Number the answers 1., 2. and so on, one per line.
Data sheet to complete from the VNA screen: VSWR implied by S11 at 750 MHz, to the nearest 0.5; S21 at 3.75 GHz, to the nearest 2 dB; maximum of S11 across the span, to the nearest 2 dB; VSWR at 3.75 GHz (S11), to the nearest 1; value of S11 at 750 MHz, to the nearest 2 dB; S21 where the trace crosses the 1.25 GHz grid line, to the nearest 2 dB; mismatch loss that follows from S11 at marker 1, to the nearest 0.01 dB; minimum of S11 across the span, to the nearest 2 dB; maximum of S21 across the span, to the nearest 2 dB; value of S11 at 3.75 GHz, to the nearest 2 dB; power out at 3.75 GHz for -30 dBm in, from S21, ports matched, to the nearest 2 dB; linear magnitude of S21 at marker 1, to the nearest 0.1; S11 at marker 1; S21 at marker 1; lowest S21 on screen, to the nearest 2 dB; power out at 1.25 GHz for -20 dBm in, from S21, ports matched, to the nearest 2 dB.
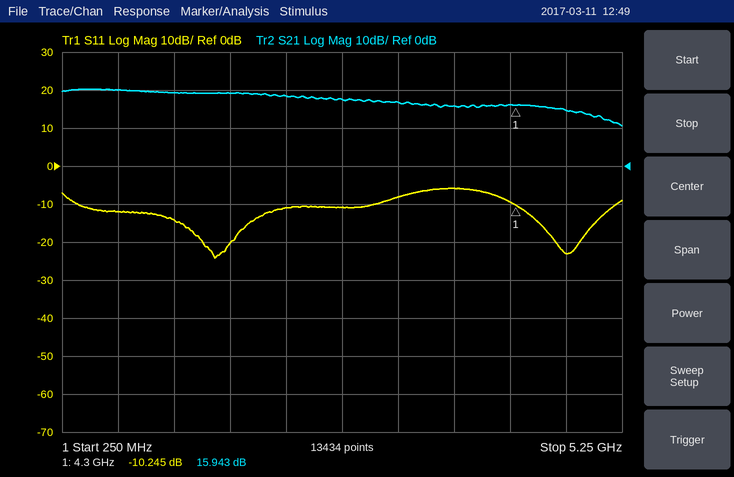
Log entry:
1. 1.5
2. 16 dB
3. -6 dB
4. 3
5. -12 dB
6. 20 dB
7. 0.43 dB
8. -24 dB
9. 20 dB
10. -6 dB
11. -14 dBm
12. 6.3
13. -10.245 dB
14. 15.943 dB
15. 10 dB
16. 0 dBm
